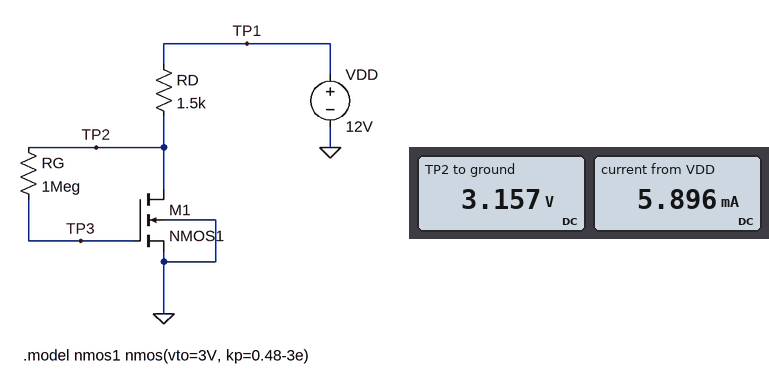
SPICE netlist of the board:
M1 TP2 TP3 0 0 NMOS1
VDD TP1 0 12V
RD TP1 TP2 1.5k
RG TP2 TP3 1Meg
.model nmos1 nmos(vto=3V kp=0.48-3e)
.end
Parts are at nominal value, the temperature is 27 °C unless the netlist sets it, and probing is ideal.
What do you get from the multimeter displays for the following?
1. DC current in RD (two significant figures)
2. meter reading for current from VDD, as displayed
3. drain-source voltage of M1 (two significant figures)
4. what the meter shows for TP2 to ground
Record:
5.9 mA
5.896 mA
3.2 V
3.157 V
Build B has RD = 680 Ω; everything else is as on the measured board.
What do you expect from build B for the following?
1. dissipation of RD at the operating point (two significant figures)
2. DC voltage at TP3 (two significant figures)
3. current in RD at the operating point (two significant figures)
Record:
110 mW
3.2 V
13 mA
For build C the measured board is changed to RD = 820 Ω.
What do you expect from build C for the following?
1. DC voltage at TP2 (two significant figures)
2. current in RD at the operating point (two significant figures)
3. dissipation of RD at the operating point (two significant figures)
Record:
3.2 V
11 mA
94 mW
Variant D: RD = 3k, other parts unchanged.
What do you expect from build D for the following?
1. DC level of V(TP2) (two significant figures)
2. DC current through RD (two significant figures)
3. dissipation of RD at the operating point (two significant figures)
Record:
3.1 V
3.0 mA
26 mW
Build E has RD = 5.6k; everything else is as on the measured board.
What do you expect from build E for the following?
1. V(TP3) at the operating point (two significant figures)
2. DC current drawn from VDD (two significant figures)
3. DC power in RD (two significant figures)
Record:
3.1 V
1.6 mA
14 mW
